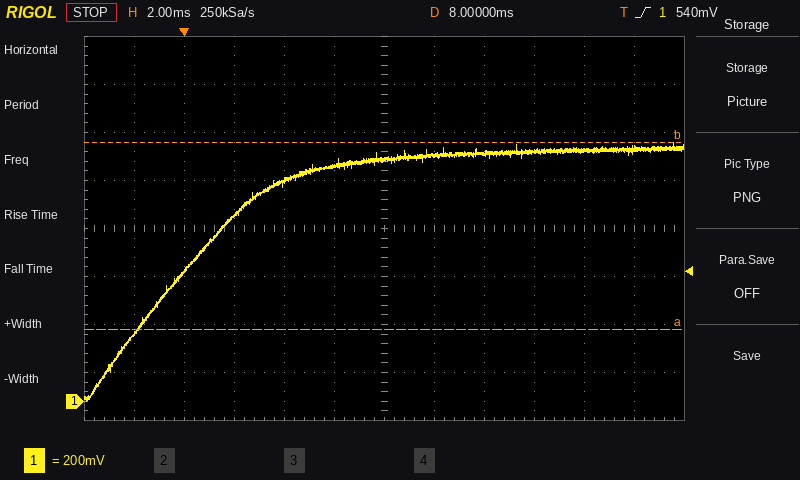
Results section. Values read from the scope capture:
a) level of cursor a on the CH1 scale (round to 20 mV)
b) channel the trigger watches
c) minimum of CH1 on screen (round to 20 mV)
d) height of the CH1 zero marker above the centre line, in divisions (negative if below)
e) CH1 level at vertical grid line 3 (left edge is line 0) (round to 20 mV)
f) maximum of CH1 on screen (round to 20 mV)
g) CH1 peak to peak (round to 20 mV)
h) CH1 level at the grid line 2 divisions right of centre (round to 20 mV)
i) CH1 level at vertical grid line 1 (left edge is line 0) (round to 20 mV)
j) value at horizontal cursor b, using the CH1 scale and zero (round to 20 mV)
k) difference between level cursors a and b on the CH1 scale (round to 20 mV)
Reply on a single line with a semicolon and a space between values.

300 mV; CH1; 0 mV; -3.6 div; 780 mV; 1.08 V; 1.08 V; 1.04 V; 280 mV; 1.08 V; 780 mV
